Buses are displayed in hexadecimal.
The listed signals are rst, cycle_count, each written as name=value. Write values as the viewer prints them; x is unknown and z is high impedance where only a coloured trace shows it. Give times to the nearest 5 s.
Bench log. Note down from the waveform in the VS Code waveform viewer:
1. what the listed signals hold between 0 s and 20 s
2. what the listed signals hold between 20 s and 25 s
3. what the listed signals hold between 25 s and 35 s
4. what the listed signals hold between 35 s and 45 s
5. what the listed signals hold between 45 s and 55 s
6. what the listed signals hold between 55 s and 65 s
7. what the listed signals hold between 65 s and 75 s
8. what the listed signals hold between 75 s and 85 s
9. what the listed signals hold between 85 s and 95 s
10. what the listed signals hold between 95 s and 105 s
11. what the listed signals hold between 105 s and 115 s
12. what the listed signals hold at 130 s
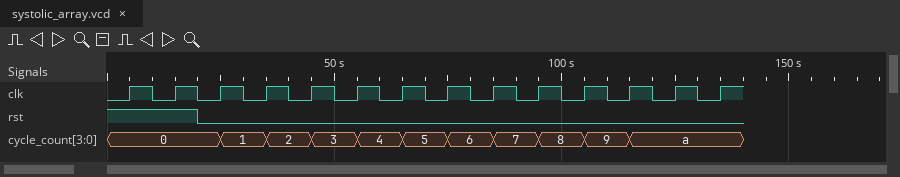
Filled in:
rst=1, cycle_count=0
rst=0, cycle_count=0
rst=0, cycle_count=1
rst=0, cycle_count=2
rst=0, cycle_count=3
rst=0, cycle_count=4
rst=0, cycle_count=5
rst=0, cycle_count=6
rst=0, cycle_count=7
rst=0, cycle_count=8
rst=0, cycle_count=9
rst=0, cycle_count=a
